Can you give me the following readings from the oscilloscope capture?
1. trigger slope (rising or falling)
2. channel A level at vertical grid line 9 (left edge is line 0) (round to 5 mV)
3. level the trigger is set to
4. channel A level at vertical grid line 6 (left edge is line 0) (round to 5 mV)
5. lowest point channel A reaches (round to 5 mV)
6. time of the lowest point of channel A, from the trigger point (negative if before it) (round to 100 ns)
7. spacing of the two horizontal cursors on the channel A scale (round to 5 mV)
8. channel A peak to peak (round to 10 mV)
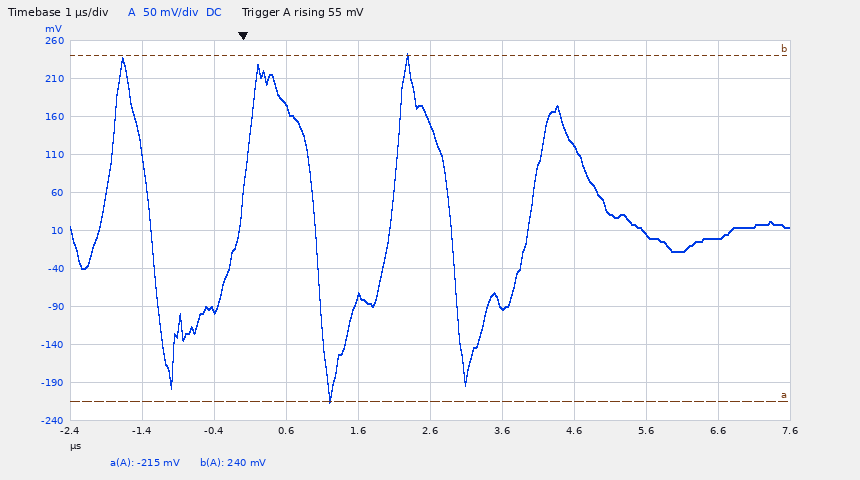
rising
0 mV
55 mV
-90 mV
-215 mV
+1.2 µs
455 mV
460 mV
